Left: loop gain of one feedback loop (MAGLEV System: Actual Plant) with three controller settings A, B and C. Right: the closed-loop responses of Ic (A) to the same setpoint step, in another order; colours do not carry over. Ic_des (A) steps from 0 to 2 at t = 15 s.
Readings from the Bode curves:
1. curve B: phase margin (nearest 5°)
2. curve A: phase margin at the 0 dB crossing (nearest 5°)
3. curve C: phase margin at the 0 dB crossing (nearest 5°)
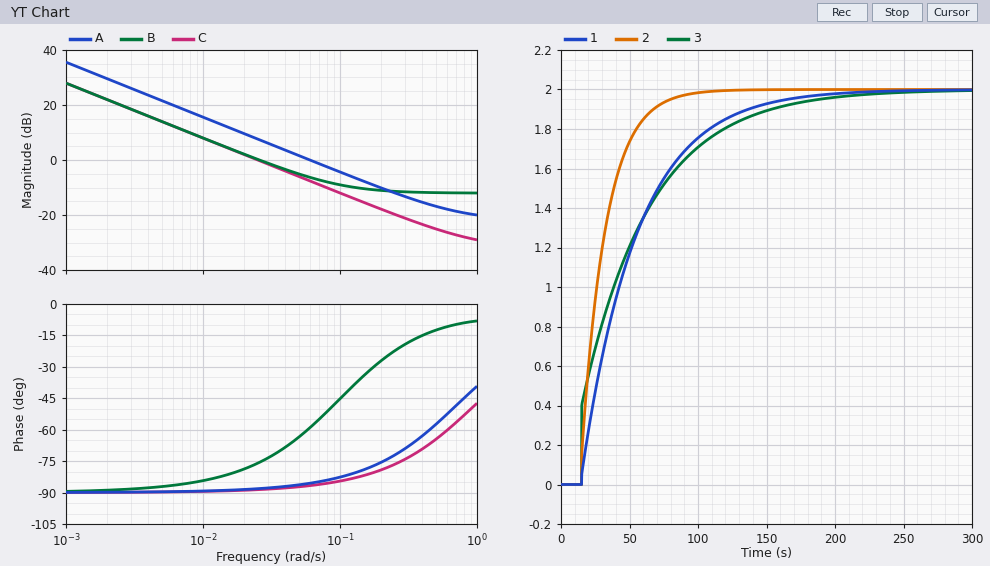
105°
95°
90°
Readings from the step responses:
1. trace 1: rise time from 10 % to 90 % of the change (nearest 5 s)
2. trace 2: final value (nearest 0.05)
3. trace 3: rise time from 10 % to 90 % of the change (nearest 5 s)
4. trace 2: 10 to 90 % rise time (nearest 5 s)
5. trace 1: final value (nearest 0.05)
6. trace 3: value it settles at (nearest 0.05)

90 s
2.00
105 s
40 s
2.00
2.00
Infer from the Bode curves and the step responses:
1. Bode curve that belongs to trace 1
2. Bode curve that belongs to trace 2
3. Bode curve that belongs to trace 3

C
A
B
